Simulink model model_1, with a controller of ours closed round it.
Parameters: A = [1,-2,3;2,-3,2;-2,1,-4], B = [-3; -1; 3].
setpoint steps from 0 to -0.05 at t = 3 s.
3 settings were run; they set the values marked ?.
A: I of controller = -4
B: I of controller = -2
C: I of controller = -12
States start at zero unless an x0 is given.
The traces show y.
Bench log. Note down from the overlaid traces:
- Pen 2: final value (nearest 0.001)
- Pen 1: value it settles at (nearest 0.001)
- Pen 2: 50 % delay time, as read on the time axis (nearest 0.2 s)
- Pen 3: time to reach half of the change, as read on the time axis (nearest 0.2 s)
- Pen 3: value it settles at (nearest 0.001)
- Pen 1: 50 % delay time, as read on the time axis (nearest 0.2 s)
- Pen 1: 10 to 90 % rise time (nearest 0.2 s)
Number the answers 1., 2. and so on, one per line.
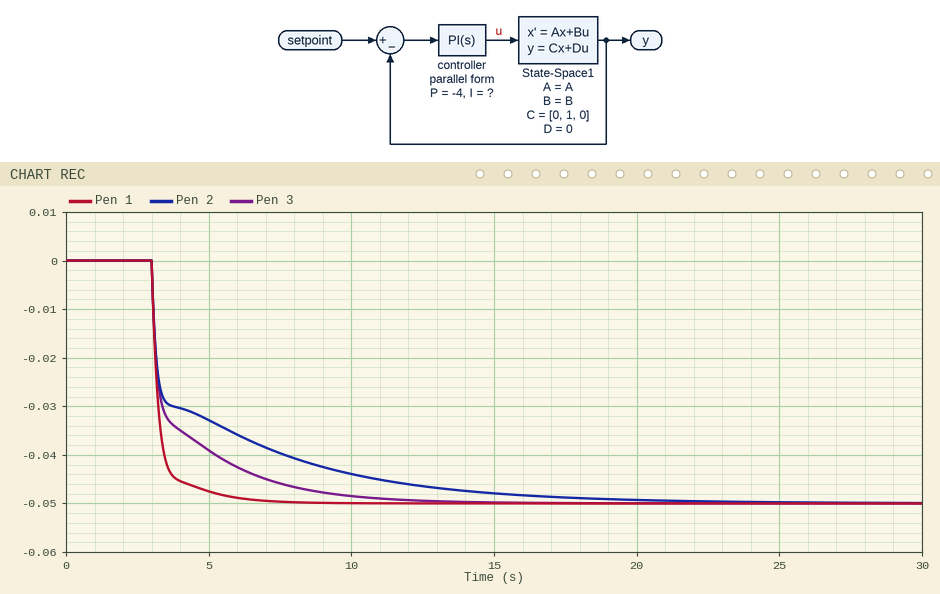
1. -0.050
2. -0.050
3. 3.2 s
4. 3.2 s
5. -0.050
6. 3.2 s
7. 0.8 s
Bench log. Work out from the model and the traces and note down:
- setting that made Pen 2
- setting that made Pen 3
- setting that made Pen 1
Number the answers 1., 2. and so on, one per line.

1. B
2. A
3. C
